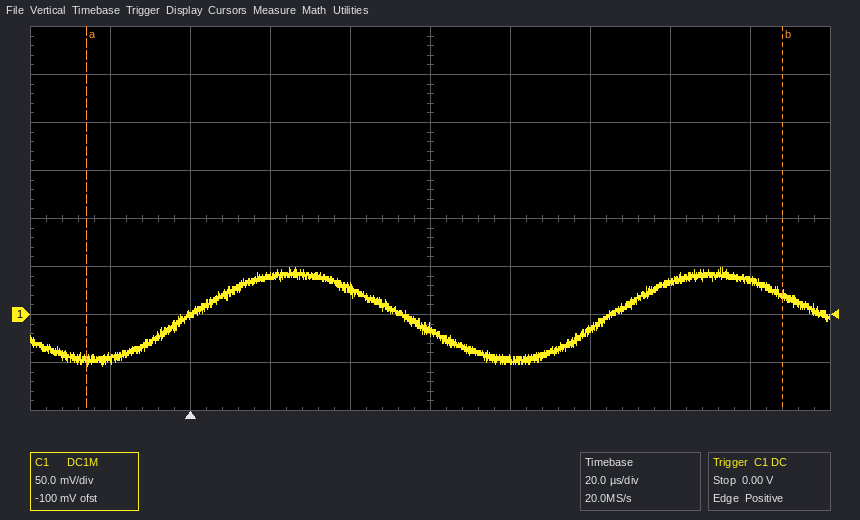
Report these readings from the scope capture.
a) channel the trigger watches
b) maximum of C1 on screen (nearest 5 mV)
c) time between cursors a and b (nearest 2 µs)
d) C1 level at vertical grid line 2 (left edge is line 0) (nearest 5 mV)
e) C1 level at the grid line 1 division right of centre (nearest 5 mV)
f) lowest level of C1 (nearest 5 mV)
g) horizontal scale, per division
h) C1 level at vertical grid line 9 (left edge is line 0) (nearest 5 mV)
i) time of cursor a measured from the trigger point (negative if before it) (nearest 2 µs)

C1
50 mV
174 µs
0 mV
-45 mV
-55 mV
20 µs
35 mV
-26 µs
